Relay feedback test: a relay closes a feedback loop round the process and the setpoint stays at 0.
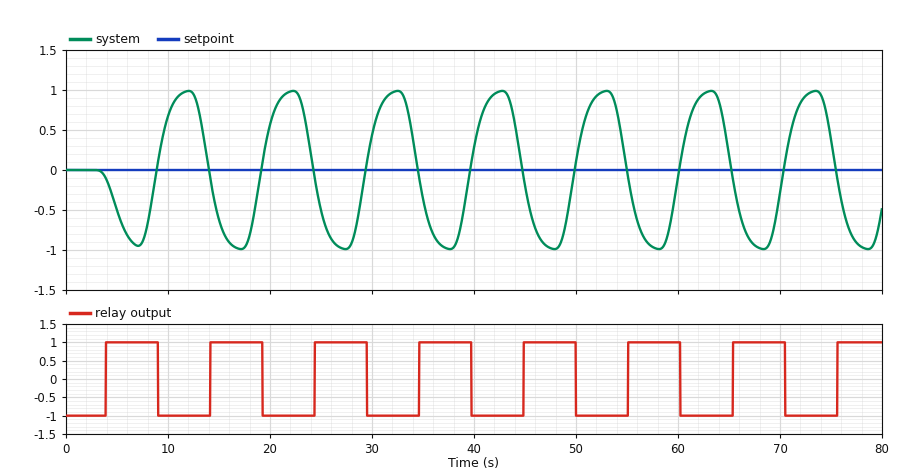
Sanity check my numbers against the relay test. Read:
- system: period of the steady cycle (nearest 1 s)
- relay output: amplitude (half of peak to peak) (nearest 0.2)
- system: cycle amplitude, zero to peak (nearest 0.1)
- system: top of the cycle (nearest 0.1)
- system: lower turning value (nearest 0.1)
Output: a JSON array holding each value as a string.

["10 s", "1.0", "1.0", "1.0", "-1.0"]
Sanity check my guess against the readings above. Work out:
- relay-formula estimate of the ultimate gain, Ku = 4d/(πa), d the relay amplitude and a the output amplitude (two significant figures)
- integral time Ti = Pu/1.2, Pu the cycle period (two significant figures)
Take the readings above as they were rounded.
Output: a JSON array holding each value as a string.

["1.3", "8.3 s"]
